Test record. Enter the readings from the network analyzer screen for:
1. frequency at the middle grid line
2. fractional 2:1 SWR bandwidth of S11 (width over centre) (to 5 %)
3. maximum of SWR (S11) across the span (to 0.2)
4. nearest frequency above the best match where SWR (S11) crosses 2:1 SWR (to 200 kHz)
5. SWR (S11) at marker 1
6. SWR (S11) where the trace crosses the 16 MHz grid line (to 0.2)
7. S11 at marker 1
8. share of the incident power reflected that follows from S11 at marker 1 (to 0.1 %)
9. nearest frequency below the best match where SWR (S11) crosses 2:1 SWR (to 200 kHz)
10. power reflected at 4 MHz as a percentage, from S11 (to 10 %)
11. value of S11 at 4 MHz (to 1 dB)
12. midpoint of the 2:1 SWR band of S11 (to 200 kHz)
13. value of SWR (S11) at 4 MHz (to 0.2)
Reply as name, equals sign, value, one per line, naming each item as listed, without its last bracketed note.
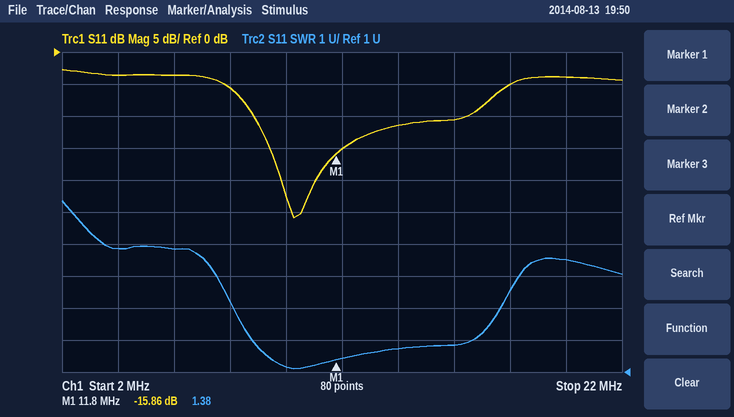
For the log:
frequency at the middle grid line = 12 MHz
fractional 2:1 SWR bandwidth of S11 (width over centre) = 60 %
maximum of SWR (S11) across the span = 6.4
nearest frequency above the best match where SWR (S11) crosses 2:1 SWR = 16.6 MHz
SWR (S11) at marker 1 = 1.38
SWR (S11) where the trace crosses the 16 MHz grid line = 1.8
S11 at marker 1 = -15.86 dB
share of the incident power reflected that follows from S11 at marker 1 = 2.6 %
nearest frequency below the best match where SWR (S11) crosses 2:1 SWR = 8.8 MHz
power reflected at 4 MHz as a percentage, from S11 = 40 %
value of S11 at 4 MHz = -4 dB
midpoint of the 2:1 SWR band of S11 = 12.8 MHz
value of SWR (S11) at 4 MHz = 4.8
